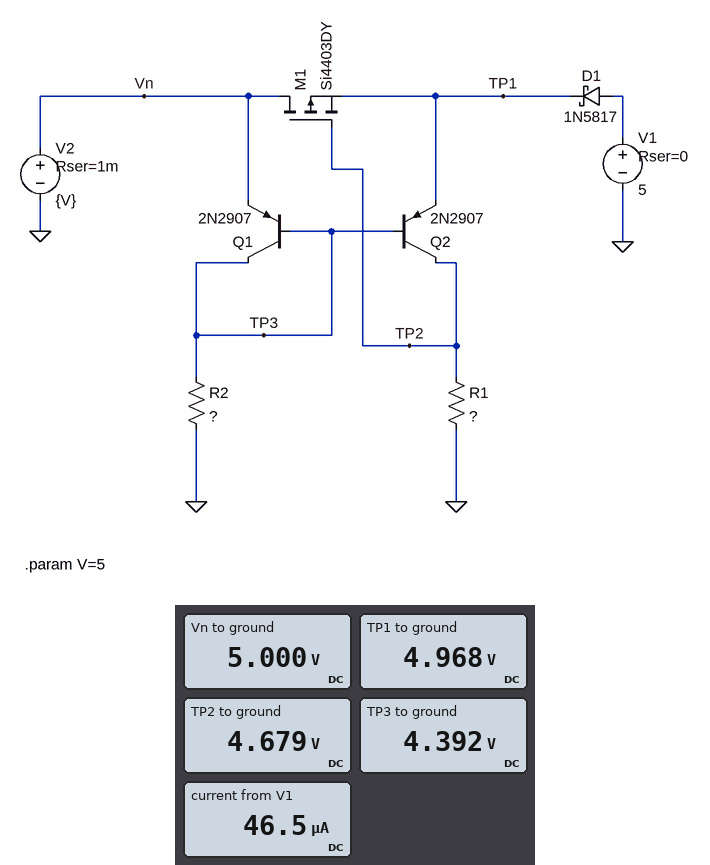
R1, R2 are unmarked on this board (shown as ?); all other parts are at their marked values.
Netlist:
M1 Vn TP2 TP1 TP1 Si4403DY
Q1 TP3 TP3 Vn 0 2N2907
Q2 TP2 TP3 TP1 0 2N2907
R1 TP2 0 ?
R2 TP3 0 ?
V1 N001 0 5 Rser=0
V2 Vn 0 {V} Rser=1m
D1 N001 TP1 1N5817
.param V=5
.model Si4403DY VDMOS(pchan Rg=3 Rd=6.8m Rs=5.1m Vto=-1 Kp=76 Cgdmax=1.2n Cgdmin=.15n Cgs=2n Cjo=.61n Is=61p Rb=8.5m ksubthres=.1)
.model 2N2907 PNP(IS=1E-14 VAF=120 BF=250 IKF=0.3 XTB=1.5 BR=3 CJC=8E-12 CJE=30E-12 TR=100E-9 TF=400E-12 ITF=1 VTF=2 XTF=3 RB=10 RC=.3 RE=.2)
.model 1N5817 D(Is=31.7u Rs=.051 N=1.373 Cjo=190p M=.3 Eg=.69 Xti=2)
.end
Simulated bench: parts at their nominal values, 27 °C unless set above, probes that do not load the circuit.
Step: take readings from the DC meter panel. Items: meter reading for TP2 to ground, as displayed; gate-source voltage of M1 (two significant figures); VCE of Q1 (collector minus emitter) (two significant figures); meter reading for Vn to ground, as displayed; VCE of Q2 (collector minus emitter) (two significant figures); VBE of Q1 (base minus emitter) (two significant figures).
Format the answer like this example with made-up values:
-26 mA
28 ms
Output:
4.679 V
-290 mV
-610 mV
5.000 V
-290 mV
-610 mV
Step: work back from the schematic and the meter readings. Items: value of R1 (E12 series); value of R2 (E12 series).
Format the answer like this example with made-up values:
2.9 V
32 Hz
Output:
100 kΩ
27 kΩ
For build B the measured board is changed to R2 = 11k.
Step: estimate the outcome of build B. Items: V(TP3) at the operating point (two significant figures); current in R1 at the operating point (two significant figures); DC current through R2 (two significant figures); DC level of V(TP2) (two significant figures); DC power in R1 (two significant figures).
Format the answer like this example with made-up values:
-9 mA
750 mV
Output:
4.4 V
49 µA
400 µA
4.9 V
240 µW
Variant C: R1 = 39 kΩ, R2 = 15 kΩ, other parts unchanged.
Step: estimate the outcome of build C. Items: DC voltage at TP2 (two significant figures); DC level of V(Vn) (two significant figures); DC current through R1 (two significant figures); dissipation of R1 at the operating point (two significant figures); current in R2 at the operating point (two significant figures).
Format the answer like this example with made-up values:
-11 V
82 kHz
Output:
4.4 V
5.0 V
110 µA
500 µW
290 µA
